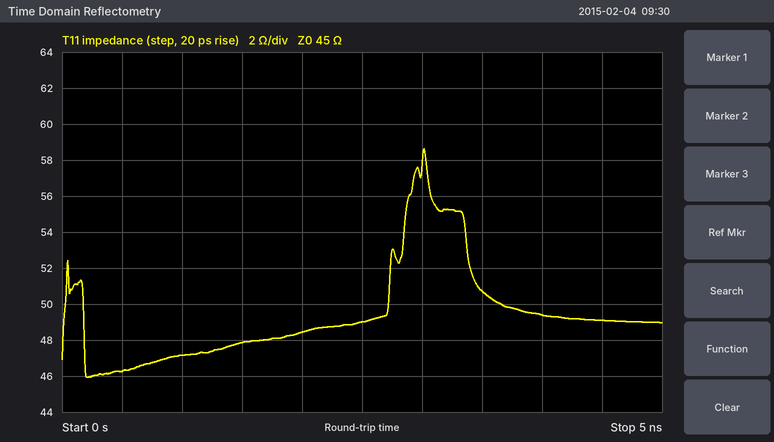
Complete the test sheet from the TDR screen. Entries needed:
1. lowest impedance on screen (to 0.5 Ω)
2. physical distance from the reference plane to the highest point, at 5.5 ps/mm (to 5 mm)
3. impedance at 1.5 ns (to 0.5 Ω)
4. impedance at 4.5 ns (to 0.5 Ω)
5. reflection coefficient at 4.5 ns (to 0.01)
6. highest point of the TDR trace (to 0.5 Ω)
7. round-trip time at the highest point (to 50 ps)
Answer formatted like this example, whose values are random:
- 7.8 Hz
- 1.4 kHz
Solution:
- 46.0 Ω
- 275 mm
- 48.0 Ω
- 49.0 Ω
- +0.04
- 58.5 Ω
- 3.00 ns
